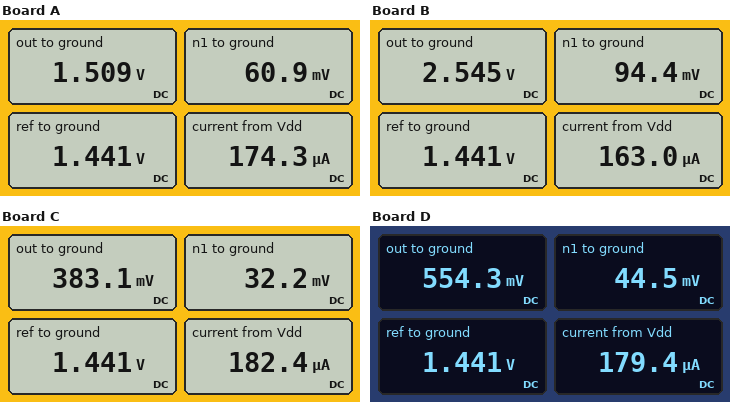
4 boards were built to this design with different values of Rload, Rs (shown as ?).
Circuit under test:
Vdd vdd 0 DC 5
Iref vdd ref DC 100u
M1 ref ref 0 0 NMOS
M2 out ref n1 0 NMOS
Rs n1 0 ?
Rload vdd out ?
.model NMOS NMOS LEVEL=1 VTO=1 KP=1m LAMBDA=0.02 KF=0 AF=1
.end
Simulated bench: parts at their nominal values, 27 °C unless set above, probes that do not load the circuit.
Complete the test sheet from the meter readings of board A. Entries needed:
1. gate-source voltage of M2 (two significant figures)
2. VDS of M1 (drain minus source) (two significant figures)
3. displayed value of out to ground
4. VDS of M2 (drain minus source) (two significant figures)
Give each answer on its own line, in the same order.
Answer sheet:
1.4 V
1.4 V
1.509 V
1.4 V
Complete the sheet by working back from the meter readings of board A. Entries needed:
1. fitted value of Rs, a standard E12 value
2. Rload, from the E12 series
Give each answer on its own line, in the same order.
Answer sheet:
820 Ω
47 kΩ
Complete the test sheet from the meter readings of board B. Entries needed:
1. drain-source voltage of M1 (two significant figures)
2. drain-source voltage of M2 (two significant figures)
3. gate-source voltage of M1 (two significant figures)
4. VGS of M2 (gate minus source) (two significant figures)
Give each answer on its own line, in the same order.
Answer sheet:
1.4 V
2.5 V
1.4 V
1.3 V
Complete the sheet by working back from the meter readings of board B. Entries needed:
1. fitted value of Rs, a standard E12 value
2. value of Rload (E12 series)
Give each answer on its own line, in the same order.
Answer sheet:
1.5 kΩ
39 kΩ
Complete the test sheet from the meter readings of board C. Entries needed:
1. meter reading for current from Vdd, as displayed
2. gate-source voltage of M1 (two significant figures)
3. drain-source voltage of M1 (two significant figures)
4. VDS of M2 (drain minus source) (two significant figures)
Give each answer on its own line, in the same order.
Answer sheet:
182.4 µA
1.4 V
1.4 V
350 mV
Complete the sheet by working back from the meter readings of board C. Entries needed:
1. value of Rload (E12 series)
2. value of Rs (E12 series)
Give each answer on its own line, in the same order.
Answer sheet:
56 kΩ
390 Ω
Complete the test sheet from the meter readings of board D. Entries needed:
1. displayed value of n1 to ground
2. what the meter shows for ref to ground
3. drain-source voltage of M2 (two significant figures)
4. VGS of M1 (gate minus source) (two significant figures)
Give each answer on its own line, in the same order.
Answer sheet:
44.5 mV
1.441 V
510 mV
1.4 V
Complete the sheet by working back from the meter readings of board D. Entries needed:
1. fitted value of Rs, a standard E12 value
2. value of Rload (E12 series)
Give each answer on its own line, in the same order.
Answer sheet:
560 Ω
56 kΩ
